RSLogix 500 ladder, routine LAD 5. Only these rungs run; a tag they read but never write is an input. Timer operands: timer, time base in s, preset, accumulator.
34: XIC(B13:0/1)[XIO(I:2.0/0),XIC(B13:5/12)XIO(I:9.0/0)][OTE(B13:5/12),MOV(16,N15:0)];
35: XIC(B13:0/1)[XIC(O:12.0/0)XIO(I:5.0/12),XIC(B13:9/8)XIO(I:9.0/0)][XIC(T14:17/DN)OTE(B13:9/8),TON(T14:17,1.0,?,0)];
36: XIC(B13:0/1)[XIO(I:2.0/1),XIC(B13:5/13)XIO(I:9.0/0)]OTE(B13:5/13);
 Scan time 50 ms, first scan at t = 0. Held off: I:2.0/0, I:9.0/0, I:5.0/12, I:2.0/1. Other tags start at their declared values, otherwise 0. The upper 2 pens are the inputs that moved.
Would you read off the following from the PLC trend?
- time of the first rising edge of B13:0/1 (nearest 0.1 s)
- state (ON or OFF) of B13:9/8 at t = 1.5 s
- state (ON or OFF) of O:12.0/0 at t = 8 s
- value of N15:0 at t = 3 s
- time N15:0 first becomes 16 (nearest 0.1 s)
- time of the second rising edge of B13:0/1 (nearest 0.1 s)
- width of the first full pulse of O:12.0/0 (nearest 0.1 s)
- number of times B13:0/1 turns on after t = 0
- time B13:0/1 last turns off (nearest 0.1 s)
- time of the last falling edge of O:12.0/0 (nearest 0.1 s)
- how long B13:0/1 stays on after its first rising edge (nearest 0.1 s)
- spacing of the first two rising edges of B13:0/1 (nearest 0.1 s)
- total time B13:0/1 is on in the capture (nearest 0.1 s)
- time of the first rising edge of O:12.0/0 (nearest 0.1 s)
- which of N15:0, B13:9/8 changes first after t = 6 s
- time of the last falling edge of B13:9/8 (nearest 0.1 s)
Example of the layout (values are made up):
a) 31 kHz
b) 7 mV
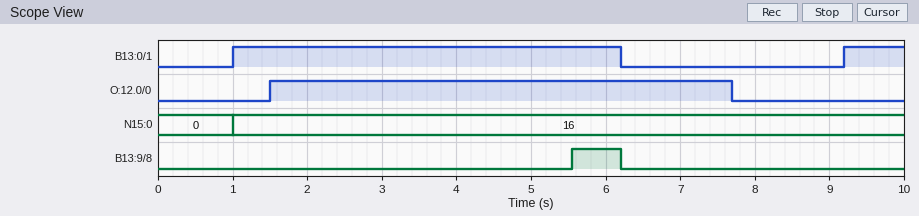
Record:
a) 1.0 s
b) OFF
c) OFF
d) 16
e) 1.0 s
f) 9.2 s
g) 6.2 s
h) 2
i) 6.2 s
j) 7.7 s
k) 5.2 s
l) 8.2 s
m) 6.0 s
n) 1.5 s
o) B13:9/8
p) 6.2 s
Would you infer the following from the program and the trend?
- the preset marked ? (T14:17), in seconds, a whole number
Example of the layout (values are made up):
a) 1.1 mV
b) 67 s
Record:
a) 4 s
